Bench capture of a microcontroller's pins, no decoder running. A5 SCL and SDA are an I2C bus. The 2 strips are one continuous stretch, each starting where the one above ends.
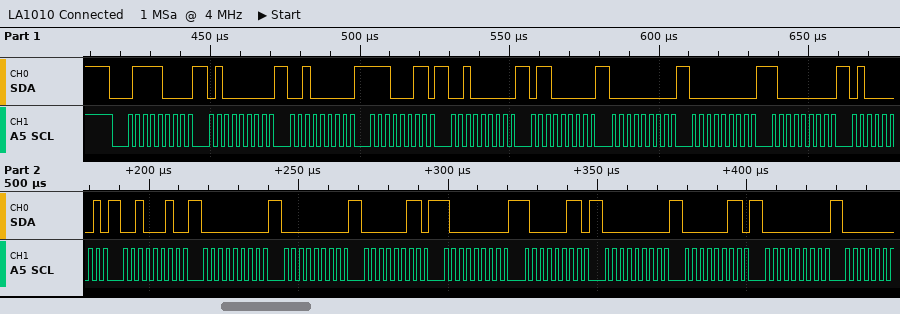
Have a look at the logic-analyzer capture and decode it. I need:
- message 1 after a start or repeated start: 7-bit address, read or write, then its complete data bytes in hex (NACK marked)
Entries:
0x3C write: 40 20 E3 20 60 00 00 80 41 22 00 00 03 80 83 00 03 00
